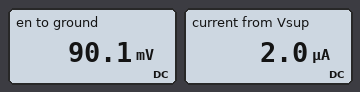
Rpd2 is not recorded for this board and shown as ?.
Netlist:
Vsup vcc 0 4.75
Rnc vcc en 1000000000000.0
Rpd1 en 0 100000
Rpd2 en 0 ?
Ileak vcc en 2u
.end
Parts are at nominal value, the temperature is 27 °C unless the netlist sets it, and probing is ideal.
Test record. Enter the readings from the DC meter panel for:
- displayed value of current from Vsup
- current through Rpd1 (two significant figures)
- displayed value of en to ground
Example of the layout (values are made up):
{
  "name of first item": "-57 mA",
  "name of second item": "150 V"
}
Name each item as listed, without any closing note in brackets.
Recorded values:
{
  "displayed value of current from Vsup": "2.0 µA",
  "current through Rpd1": "900 nA",
  "displayed value of en to ground": "90.1 mV"
}
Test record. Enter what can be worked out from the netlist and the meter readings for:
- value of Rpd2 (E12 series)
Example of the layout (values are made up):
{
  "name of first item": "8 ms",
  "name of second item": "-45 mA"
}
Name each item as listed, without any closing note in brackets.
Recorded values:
{
  "value of Rpd2": "82 kΩ"
}
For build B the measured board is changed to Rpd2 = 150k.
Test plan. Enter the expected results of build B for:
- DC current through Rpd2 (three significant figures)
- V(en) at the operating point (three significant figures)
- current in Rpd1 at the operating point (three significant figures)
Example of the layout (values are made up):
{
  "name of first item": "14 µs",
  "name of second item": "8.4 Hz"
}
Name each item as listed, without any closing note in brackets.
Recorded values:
{
  "DC current through Rpd2": "800 nA",
  "V(en) at the operating point": "120 mV",
  "current in Rpd1 at the operating point": "1.20 µA"
}
